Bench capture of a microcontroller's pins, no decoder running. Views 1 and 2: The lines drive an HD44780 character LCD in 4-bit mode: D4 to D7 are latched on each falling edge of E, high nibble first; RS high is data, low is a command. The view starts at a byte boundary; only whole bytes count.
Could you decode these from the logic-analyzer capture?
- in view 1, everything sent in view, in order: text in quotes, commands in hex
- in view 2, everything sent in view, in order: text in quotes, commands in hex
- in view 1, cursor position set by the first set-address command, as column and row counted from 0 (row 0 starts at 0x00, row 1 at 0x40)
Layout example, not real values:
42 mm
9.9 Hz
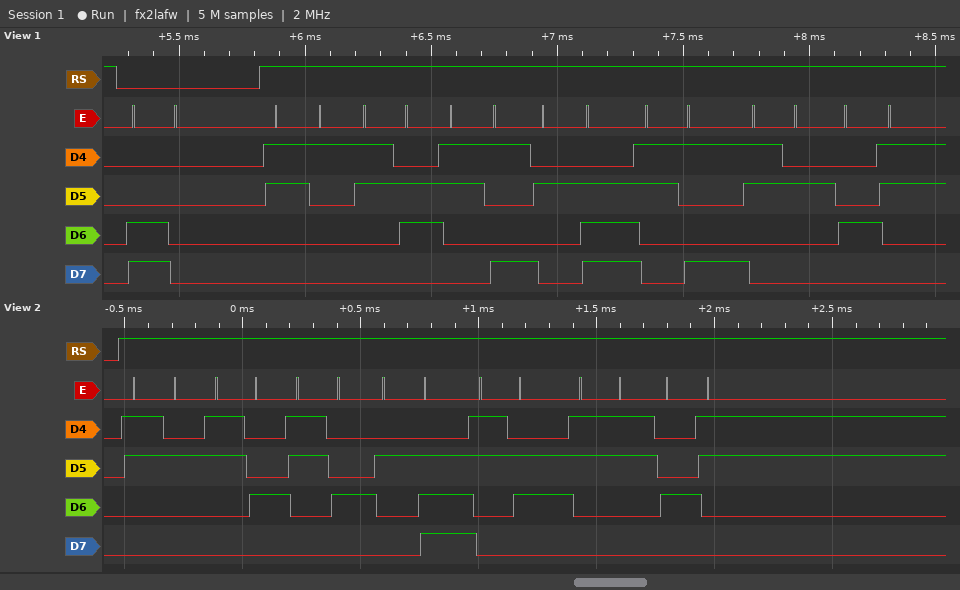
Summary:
0xC0 "169.92C"
"244.63C"
column 0, row 1
